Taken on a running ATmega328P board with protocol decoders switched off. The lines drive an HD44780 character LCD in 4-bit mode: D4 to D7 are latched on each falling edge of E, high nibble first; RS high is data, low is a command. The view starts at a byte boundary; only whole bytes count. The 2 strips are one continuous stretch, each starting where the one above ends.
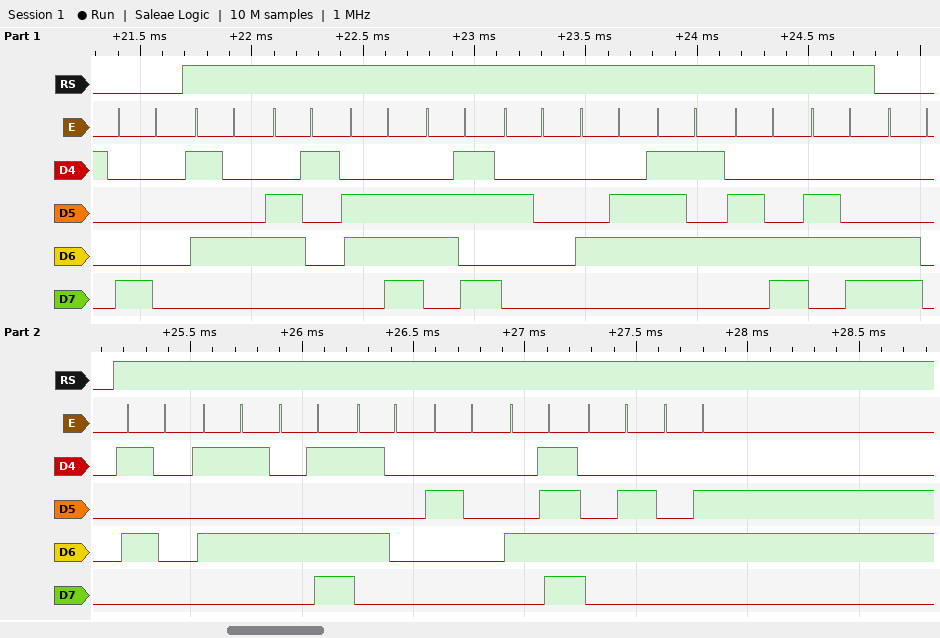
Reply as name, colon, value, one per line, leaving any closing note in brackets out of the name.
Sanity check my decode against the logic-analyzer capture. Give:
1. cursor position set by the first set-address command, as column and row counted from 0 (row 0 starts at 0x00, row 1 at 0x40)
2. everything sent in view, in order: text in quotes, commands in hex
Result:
cursor position set by the first set-address command, as column and row counted from 0: column 0, row 0
everything sent in view, in order: text in quotes, commands in hex: 0x80 "Tank Full" 0xC0 "PUMP OFF"
